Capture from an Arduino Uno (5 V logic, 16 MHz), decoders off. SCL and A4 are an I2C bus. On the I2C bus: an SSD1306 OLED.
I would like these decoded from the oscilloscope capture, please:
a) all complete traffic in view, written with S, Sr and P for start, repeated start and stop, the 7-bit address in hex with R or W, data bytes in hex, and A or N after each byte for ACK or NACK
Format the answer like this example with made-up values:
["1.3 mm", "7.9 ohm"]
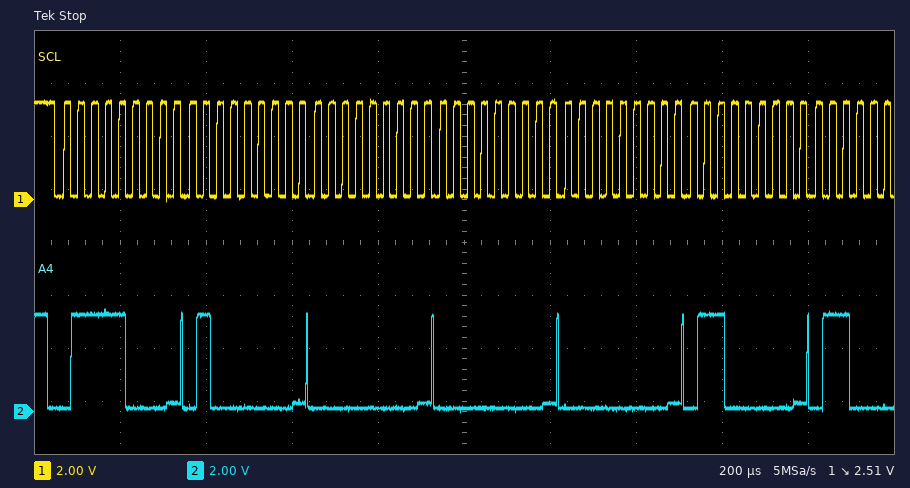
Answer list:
["S 3CW A 40 A 00 A 00 A 00 A 60 A"]
